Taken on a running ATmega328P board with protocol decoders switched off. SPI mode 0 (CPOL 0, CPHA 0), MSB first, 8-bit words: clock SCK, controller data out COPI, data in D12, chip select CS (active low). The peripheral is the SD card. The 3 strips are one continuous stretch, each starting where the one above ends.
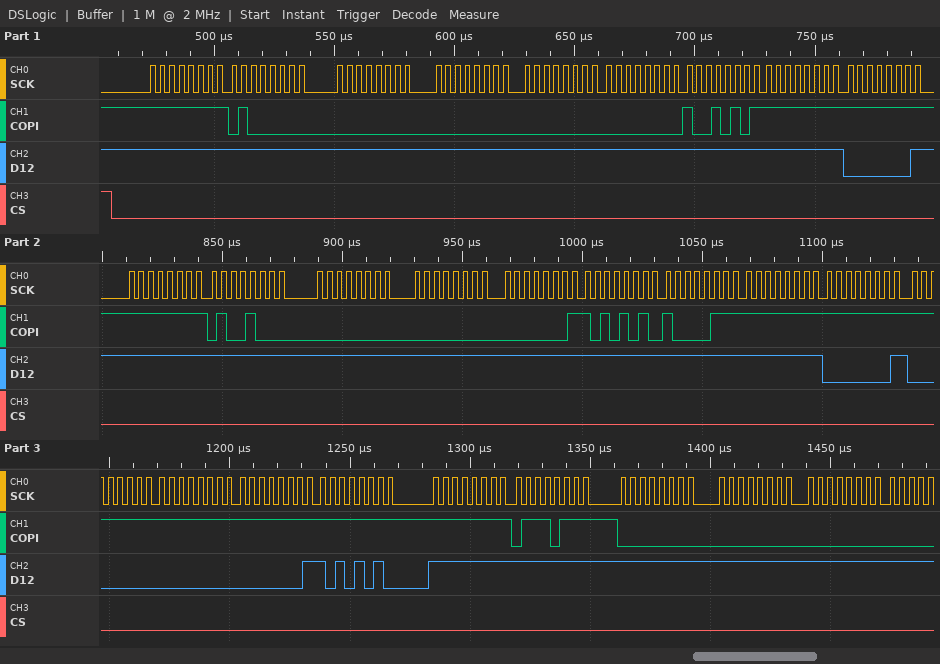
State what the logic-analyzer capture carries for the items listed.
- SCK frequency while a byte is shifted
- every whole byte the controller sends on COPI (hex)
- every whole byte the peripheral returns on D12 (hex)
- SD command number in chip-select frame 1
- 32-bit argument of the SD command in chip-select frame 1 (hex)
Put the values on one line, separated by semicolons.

250 kHz; 0xFF 0x40 0x00 0x00 0x00 0x00 0x95 0xFF 0xFF 0xFF 0x48 0x00 0x00 0x01 0xAA 0x87 0xFF 0xFF 0xFF 0xFF 0xFF 0xFF 0xFF 0x77 0x00 0x00 0x00; 0xFF 0xFF 0xFF 0xFF 0xFF 0xFF 0xFF 0xFF 0x01 0xFF 0xFF 0xFF 0xFF 0xFF 0xFF 0xFF 0xFF 0x01 0x00 0x00 0x01 0xAA 0xFF 0xFF 0xFF 0xFF 0xFF; CMD0; 0x00000000
